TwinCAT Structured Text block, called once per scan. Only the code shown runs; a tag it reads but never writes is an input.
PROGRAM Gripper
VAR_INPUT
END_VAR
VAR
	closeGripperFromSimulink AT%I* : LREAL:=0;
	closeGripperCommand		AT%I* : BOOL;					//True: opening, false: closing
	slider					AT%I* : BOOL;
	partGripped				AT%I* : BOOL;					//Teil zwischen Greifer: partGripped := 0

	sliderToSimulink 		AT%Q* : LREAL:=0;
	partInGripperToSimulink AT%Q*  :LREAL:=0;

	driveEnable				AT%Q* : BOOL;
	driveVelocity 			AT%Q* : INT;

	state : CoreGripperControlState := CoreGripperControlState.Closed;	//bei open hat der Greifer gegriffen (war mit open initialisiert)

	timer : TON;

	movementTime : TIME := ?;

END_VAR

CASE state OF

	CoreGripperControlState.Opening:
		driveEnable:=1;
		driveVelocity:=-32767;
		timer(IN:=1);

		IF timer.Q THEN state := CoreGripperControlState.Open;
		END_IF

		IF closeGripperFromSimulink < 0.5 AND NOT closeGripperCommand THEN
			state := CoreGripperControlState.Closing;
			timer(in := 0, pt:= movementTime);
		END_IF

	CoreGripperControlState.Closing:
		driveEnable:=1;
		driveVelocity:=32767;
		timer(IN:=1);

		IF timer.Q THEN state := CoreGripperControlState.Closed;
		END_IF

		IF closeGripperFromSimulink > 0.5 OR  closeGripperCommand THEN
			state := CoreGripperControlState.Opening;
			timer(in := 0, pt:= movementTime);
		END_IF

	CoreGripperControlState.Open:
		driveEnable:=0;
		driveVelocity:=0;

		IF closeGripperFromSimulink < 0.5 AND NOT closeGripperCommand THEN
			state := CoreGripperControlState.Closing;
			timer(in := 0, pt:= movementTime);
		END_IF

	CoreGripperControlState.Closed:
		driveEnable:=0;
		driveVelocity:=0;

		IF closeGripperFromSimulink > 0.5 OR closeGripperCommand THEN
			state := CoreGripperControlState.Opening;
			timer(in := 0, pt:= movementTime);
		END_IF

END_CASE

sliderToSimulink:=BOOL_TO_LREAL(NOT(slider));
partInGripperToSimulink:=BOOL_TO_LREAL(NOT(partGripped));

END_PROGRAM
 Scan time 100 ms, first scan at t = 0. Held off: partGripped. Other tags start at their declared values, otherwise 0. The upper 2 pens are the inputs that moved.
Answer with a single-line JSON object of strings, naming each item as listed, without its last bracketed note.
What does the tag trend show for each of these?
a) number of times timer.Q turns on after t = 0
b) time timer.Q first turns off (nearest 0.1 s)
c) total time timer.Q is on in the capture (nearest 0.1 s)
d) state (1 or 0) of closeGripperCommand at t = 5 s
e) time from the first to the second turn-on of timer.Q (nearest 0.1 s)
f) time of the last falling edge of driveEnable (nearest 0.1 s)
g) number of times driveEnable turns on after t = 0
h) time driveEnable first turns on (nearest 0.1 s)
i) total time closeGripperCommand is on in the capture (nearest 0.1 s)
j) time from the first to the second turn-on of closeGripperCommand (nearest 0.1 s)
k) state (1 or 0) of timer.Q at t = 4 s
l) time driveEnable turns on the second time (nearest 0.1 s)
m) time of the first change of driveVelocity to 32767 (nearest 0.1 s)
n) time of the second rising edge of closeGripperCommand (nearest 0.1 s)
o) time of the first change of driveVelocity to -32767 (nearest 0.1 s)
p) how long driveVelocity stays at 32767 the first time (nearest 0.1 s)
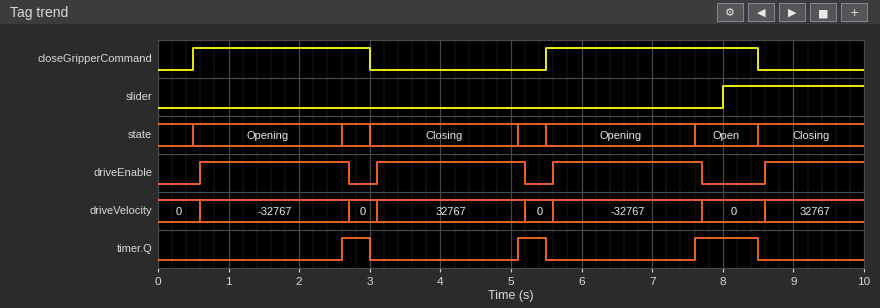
{"number of times timer.Q turns on after t = 0": "3", "time timer.Q first turns off": "3.0 s", "total time timer.Q is on in the capture": "1.7 s", "state (1 or 0) of closeGripperCommand at t = 5 s": "0", "time from the first to the second turn-on of timer.Q": "2.5 s", "time of the last falling edge of driveEnable": "7.7 s", "number of times driveEnable turns on after t = 0": "4", "time driveEnable first turns on": "0.6 s", "total time closeGripperCommand is on in the capture": "5.5 s", "time from the first to the second turn-on of closeGripperCommand": "5.0 s", "state (1 or 0) of timer.Q at t = 4 s": "0", "time driveEnable turns on the second time": "3.1 s", "time of the first change of driveVelocity to 32767": "3.1 s", "time of the second rising edge of closeGripperCommand": "5.5 s", "time of the first change of driveVelocity to -32767": "0.6 s", "how long driveVelocity stays at 32767 the first time": "2.1 s"}
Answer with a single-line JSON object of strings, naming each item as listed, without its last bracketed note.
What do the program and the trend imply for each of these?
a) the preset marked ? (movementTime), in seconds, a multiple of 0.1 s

{"the preset marked ? (movementTime), in seconds, a multiple of 0.1 s": "2.0 s"}
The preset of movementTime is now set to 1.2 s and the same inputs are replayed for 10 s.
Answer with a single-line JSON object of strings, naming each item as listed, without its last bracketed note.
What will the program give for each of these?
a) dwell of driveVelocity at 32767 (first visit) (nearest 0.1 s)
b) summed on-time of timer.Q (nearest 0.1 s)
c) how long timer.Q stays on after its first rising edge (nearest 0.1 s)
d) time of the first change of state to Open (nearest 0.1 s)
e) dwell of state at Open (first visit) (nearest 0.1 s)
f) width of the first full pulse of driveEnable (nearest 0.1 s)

{"dwell of driveVelocity at 32767 (first visit)": "1.3 s", "summed on-time of timer.Q": "4.3 s", "how long timer.Q stays on after its first rising edge": "1.2 s", "time of the first change of state to Open": "1.8 s", "dwell of state at Open (first visit)": "1.2 s", "width of the first full pulse of driveEnable": "1.3 s"}
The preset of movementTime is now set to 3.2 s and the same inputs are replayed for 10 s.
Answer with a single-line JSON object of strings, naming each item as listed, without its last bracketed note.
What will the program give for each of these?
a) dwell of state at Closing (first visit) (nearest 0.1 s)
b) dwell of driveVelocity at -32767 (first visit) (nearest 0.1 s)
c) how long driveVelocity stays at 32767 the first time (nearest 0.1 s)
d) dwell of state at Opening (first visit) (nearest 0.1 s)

{"dwell of state at Closing (first visit)": "2.5 s", "dwell of driveVelocity at -32767 (first visit)": "2.5 s", "how long driveVelocity stays at 32767 the first time": "2.5 s", "dwell of state at Opening (first visit)": "2.5 s"}
